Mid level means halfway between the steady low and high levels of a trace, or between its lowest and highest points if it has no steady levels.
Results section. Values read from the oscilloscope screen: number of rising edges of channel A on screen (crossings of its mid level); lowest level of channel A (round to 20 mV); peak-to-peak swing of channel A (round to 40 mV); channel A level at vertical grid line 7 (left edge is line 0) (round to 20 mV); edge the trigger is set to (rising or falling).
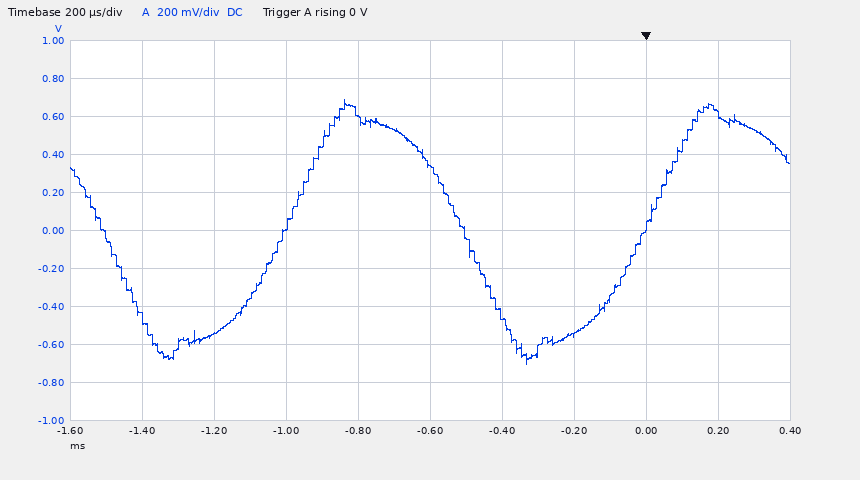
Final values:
2
-700 mV
1.40 V
-540 mV
rising
